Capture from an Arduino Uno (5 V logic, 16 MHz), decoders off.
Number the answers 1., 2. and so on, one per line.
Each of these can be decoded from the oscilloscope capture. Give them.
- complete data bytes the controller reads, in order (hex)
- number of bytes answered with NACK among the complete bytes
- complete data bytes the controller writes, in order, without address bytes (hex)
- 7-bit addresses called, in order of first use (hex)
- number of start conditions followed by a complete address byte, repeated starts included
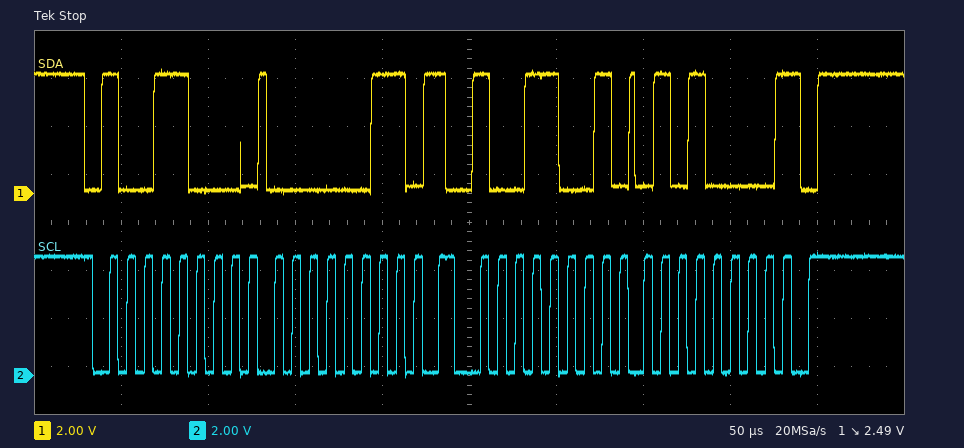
1. 50
2. 1
3. 03
4. 0x4C
5. 2
